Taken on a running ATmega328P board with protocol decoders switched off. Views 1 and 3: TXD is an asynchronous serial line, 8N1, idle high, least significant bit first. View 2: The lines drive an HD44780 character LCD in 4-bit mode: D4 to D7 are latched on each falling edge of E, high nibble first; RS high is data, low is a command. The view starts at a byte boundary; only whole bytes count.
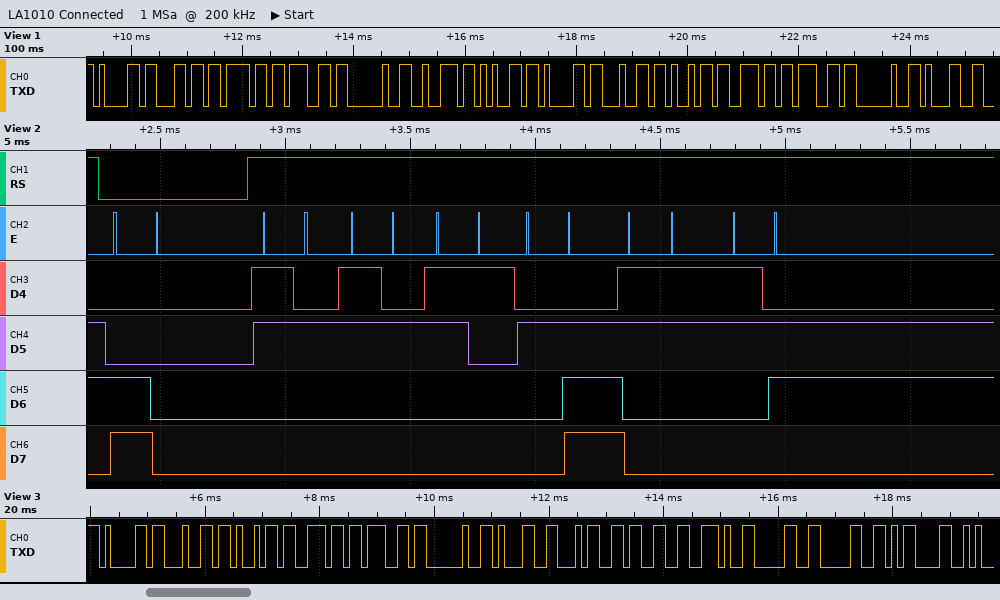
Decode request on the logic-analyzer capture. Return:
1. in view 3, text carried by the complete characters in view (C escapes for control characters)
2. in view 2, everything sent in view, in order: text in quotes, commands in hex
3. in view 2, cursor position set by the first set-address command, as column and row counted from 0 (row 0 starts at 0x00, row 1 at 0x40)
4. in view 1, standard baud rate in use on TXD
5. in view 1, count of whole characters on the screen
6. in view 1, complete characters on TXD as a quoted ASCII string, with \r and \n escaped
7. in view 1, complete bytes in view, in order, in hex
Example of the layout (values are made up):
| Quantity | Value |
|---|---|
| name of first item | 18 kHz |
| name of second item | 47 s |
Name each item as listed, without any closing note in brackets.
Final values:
| Quantity | Value |
|---|---|
| in view 3, text carried by the complete characters in view | "ading 143.00\r" |
| in view 2, everything sent in view, in order: text in quotes, commands in hex | 0xC0 "221.36" |
| in view 2, cursor position set by the first set-address command, as column and row counted from 0 | column 0, row 1 |
| in view 1, standard baud rate in use on TXD | 9600 baud |
| in view 1, count of whole characters on the screen | 14 |
| in view 1, complete characters on TXD as a quoted ASCII string, with \r and \n escaped | "alog reading 1" |
| in view 1, complete bytes in view, in order, in hex | 0x61 0x6C 0x6F 0x67 0x20 0x72 0x65 0x61 0x64 0x69 0x6E 0x67 0x20 0x31 |
